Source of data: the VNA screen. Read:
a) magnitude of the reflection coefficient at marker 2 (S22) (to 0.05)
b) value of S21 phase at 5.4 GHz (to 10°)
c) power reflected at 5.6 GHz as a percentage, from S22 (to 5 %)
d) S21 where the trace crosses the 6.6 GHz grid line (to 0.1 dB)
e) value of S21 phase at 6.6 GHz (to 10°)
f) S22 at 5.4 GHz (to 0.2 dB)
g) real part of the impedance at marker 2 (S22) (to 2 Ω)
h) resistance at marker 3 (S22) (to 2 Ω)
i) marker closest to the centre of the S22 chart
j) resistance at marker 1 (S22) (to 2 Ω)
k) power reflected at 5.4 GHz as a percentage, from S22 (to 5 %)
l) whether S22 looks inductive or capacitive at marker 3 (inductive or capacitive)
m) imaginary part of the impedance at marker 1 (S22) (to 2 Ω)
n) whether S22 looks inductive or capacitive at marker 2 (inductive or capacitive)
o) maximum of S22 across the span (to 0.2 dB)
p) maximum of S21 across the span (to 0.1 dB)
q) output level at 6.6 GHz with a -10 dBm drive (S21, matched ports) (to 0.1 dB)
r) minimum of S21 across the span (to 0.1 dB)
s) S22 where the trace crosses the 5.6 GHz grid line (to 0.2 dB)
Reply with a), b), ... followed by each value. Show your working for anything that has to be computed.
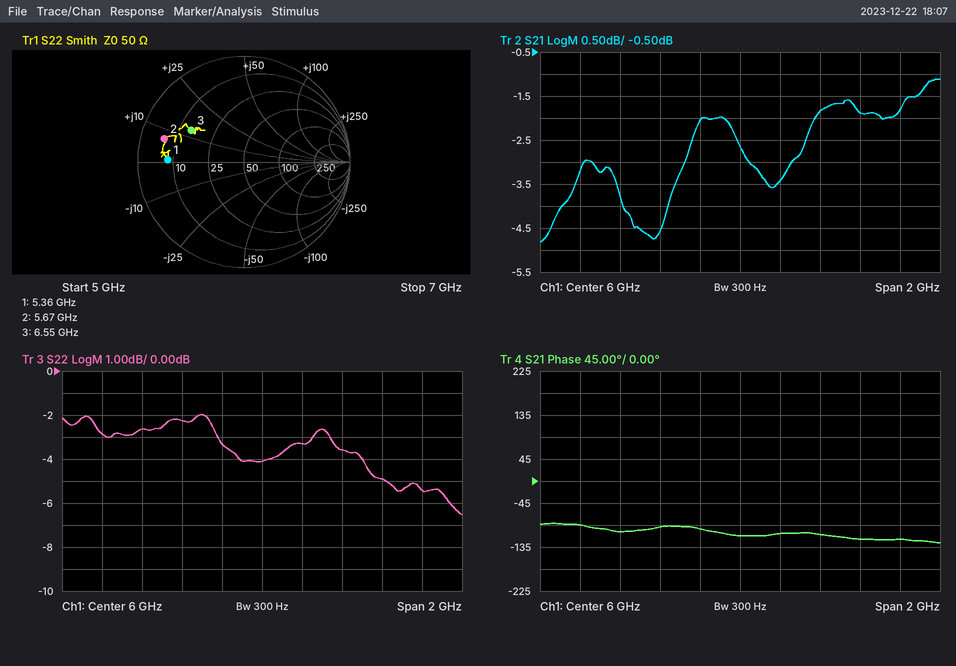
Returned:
a) 0.80
b) -100°
c) 10^(-2.2/10) ≈ 60 %
d) -1.9 dB
e) -120°
f) -2.6 dB
g) 6 Ω
h) 14 Ω
i) marker 3
j) 8 Ω
k) 10^(-2.6/10) ≈ 55 %
l) inductive
m) 0 Ω
n) inductive
o) -2.0 dB
p) -1.1 dB
q) -10 dBm + (-1.9 dB) = -11.9 dBm
r) -4.8 dB
s) -2.2 dB
